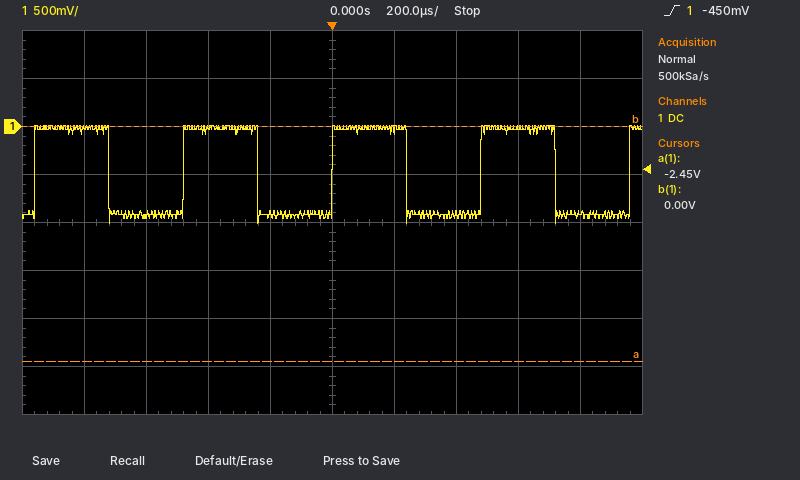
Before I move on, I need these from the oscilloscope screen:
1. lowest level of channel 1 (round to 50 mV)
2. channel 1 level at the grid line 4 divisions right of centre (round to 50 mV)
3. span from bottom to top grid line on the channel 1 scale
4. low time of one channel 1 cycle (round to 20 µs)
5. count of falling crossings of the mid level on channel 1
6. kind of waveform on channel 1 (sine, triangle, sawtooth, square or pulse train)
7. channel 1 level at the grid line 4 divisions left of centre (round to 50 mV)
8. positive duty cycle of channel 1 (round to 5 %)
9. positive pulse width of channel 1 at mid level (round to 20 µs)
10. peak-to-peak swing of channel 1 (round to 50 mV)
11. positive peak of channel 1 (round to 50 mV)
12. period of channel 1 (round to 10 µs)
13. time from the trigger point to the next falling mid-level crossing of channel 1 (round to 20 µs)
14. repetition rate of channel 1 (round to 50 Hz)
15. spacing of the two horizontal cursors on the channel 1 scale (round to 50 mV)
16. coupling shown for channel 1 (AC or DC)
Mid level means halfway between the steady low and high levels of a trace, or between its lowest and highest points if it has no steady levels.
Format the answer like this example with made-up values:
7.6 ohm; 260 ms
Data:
-1.00 V; -900 mV; 4 V; 240 µs; 4; square; -50 mV; 50 %; 240 µs; 1.00 V; 0 mV; 480 µs; 240 µs; 2.10 kHz; 2.45 V; DC
